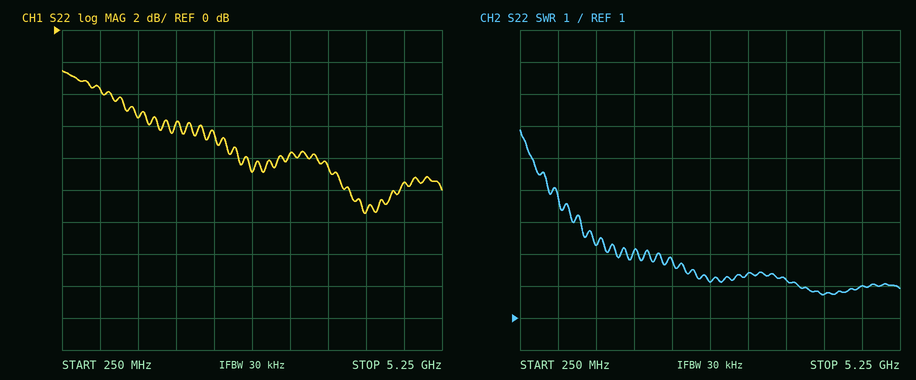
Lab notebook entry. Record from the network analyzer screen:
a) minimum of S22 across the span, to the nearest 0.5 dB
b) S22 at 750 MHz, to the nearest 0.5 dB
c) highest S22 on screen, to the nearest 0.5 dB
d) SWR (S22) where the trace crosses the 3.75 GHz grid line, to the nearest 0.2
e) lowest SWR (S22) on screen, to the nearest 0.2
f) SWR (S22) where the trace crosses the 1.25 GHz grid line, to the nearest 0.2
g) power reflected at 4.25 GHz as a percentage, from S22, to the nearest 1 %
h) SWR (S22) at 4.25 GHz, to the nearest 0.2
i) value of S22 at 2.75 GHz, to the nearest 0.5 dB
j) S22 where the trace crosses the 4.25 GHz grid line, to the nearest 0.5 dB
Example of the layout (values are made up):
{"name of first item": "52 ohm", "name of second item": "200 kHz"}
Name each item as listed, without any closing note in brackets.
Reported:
{"minimum of S22 across the span, to the nearest 0.5 dB": "-11.5 dB", "S22 at 750 MHz, to the nearest 0.5 dB": "-3.5 dB", "highest S22 on screen, to the nearest 0.5 dB": "-2.5 dB", "SWR (S22) where the trace crosses the 3.75 GHz grid line, to the nearest 0.2": "2.2", "lowest SWR (S22) on screen, to the nearest 0.2": "1.8", "SWR (S22) where the trace crosses the 1.25 GHz grid line, to the nearest 0.2": "3.2", "power reflected at 4.25 GHz as a percentage, from S22, to the nearest 1 %": "7 %", "SWR (S22) at 4.25 GHz, to the nearest 0.2": "1.8", "value of S22 at 2.75 GHz, to the nearest 0.5 dB": "-9.0 dB", "S22 where the trace crosses the 4.25 GHz grid line, to the nearest 0.5 dB": "-11.5 dB"}
